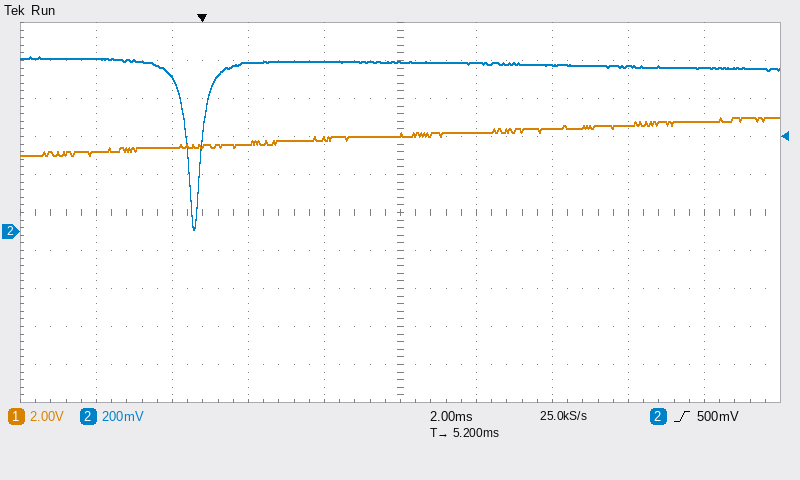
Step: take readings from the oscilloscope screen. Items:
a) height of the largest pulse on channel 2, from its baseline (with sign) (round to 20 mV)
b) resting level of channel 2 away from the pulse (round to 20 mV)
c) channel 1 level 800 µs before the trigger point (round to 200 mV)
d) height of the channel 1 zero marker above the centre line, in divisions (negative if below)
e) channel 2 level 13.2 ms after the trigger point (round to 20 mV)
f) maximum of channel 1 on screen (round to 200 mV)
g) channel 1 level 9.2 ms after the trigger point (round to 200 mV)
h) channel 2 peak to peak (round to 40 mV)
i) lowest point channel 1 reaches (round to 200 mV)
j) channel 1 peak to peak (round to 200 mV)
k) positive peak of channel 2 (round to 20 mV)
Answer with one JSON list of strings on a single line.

["-880 mV", "880 mV", "4.4 V", "-0.5 div", "860 mV", "6.0 V", "5.4 V", "920 mV", "4.0 V", "2.0 V", "920 mV"]
